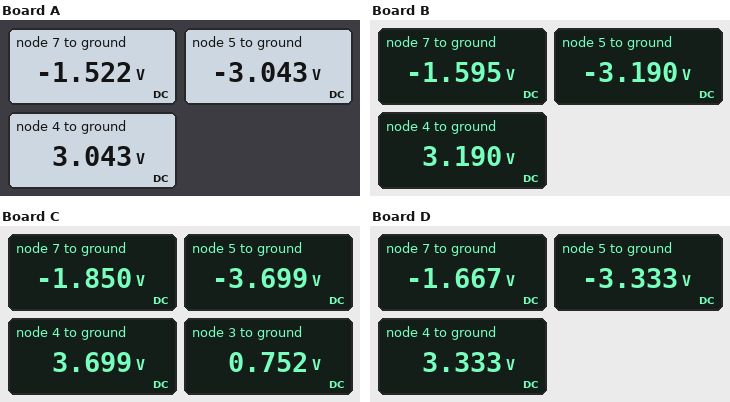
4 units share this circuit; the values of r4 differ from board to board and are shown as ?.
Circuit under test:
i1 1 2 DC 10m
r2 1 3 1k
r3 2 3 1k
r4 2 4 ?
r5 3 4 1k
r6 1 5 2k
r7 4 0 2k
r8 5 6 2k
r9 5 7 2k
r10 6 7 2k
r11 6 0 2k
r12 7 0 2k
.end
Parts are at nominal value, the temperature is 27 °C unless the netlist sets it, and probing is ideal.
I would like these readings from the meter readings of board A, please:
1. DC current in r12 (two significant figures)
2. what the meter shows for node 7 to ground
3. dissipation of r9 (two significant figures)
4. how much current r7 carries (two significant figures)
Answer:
760 µA
-1.522 V
1.2 mW
1.5 mA
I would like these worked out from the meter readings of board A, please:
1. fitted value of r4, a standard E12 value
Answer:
3.3 kΩ
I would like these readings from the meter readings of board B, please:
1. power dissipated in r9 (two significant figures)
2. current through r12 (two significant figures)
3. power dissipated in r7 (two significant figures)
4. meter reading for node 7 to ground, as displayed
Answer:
1.3 mW
800 µA
5.1 mW
-1.595 V
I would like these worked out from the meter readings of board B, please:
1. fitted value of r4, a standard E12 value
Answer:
2.2 kΩ
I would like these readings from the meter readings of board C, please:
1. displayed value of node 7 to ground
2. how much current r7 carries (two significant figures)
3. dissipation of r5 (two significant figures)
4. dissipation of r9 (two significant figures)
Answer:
-1.850 V
1.8 mA
8.7 mW
1.7 mW
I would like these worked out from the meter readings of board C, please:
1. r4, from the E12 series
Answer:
470 Ω
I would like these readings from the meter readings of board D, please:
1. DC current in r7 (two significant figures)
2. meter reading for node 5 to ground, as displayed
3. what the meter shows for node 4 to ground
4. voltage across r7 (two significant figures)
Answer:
1.7 mA
-3.333 V
3.333 V
3.3 V
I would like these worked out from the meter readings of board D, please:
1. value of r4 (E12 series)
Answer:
1.5 kΩ
